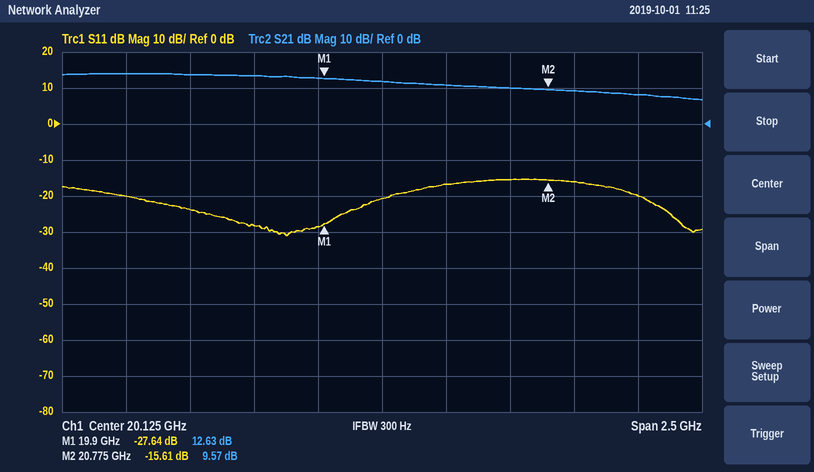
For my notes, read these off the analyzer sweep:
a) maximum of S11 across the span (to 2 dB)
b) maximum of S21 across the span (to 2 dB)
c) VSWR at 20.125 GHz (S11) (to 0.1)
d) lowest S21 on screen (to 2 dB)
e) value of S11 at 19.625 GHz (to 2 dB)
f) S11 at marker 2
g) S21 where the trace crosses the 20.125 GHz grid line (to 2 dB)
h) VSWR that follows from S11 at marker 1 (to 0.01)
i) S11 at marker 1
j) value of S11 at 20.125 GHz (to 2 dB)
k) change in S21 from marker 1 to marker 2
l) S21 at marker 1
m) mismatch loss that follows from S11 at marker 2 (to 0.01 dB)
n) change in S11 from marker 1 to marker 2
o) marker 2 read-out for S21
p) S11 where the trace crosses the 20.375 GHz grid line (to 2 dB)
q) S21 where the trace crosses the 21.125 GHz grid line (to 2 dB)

-16 dB
14 dB
1.2
6 dB
-28 dB
-15.61 dB
12 dB
1.09
-27.64 dB
-20 dB
-3.06 dB
12.63 dB
0.12 dB
12.03 dB
9.57 dB
-16 dB
8 dB
